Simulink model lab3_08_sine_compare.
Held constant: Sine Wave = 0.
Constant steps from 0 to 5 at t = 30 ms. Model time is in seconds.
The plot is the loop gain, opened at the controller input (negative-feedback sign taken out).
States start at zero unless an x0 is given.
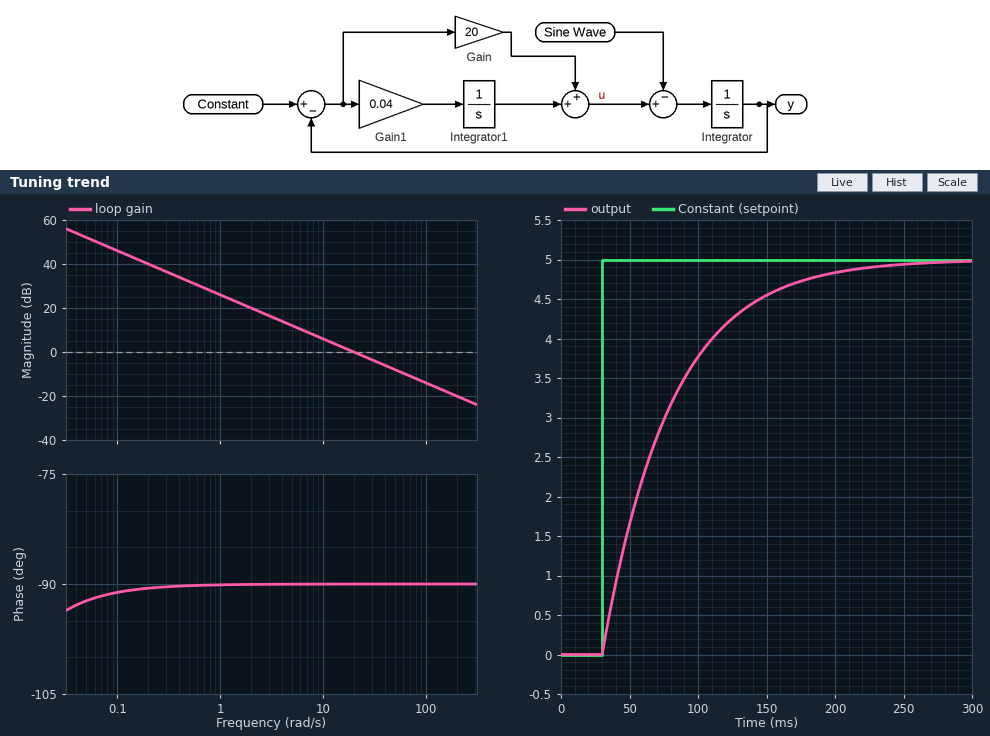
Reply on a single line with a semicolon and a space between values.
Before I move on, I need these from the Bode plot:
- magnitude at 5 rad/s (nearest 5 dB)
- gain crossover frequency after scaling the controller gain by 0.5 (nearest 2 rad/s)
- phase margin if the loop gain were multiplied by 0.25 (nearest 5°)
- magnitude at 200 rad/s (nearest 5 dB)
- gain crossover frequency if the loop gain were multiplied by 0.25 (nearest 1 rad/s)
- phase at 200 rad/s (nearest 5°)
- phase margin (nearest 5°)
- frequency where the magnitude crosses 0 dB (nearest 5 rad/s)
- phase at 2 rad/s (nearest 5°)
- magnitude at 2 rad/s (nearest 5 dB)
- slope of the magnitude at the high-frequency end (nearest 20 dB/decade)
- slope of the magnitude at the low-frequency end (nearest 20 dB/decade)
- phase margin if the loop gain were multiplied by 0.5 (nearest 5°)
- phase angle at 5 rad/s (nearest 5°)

10 dB; 10 rad/s; 90°; -20 dB; 5 rad/s; -90°; 90°; 20 rad/s; -90°; 20 dB; -20 dB/decade; -20 dB/decade; 90°; -90°
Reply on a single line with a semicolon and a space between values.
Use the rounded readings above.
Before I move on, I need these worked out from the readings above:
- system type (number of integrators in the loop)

1
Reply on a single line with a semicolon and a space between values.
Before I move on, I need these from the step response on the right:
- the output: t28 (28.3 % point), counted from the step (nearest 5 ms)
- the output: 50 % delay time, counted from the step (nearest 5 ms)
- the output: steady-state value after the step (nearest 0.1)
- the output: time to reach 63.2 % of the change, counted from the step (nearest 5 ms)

15 ms; 35 ms; 5.0; 50 ms
